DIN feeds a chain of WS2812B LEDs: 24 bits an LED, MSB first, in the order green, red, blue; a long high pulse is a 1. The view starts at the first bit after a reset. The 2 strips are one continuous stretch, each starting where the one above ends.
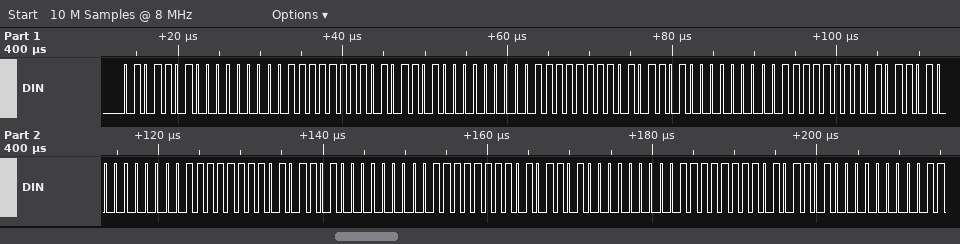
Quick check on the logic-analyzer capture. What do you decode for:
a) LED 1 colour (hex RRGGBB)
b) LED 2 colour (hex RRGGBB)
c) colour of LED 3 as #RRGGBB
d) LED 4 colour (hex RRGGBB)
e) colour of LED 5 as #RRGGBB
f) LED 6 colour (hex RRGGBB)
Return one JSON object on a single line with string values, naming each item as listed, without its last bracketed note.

{"LED 1 colour": "#005AFF", "LED 2 colour": "#005AFF", "colour of LED 3 as #RRGGBB": "#005AFF", "LED 4 colour": "#005AFF", "colour of LED 5 as #RRGGBB": "#005AFF", "LED 6 colour": "#005AFF"}
